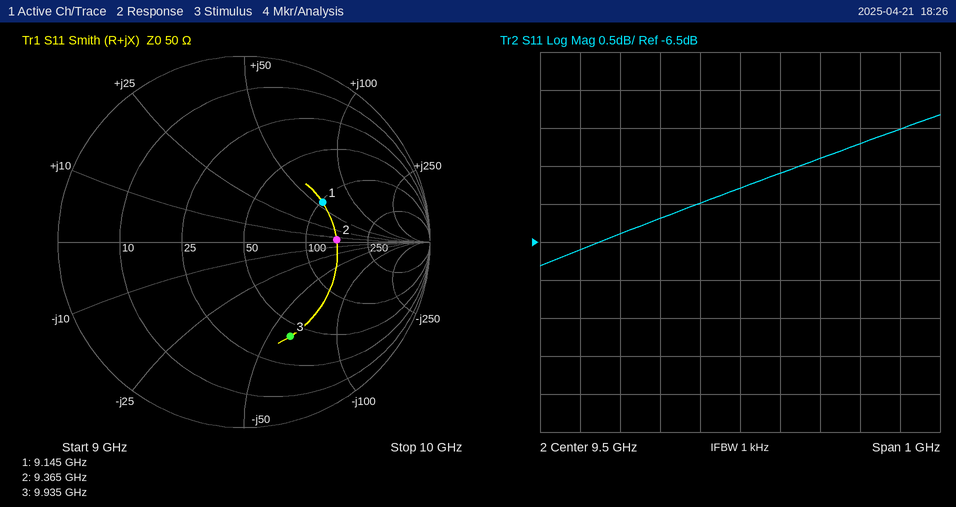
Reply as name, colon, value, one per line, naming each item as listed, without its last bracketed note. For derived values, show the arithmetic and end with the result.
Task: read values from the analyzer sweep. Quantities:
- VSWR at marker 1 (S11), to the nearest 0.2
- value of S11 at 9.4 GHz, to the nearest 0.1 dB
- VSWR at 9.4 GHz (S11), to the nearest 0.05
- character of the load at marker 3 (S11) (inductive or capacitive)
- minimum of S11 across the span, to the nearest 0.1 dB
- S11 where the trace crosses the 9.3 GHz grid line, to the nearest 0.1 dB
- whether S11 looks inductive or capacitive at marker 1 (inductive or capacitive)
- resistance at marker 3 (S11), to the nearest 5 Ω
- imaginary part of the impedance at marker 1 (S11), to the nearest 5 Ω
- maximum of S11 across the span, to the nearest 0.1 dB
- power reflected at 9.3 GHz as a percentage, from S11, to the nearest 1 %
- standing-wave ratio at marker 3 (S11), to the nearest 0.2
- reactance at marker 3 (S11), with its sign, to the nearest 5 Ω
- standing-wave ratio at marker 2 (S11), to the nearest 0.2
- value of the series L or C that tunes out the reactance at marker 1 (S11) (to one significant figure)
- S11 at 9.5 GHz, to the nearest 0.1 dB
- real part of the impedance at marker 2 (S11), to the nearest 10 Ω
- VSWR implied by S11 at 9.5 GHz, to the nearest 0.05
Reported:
VSWR at marker 1 (S11), to the nearest 0.2: 2.8
value of S11 at 9.4 GHz, to the nearest 0.1 dB: -6.0 dB
VSWR at 9.4 GHz (S11), to the nearest 0.05: |Γ| = 10^(-6/20) = 0.5012; VSWR = (1 + 0.5012)/(1 − 0.5012) ≈ 3.01, so 3.00 to the nearest 0.05
character of the load at marker 3 (S11): capacitive
minimum of S11 across the span, to the nearest 0.1 dB: -6.8 dB
S11 where the trace crosses the 9.3 GHz grid line, to the nearest 0.1 dB: -6.2 dB
whether S11 looks inductive or capacitive at marker 1: inductive
resistance at marker 3 (S11), to the nearest 5 Ω: 40 Ω
imaginary part of the impedance at marker 1 (S11), to the nearest 5 Ω: +55 Ω
maximum of S11 across the span, to the nearest 0.1 dB: -4.8 dB
power reflected at 9.3 GHz as a percentage, from S11, to the nearest 1 %: 10^(-6.2/10) ≈ 24 %
standing-wave ratio at marker 3 (S11), to the nearest 0.2: 3.6
reactance at marker 3 (S11), with its sign, to the nearest 5 Ω: -60 Ω
standing-wave ratio at marker 2 (S11), to the nearest 0.2: 3.0
value of the series L or C that tunes out the reactance at marker 1 (S11): C = 1/(2π × 9.145 GHz × 55 Ω) ≈ 316 fF, so 300 fF to one significant figure
S11 at 9.5 GHz, to the nearest 0.1 dB: -5.8 dB
real part of the impedance at marker 2 (S11), to the nearest 10 Ω: 150 Ω
VSWR implied by S11 at 9.5 GHz, to the nearest 0.05: |Γ| = 10^(-5.8/20) = 0.5129; VSWR = (1 + 0.5129)/(1 − 0.5129) ≈ 3.11, so 3.10 to the nearest 0.05
